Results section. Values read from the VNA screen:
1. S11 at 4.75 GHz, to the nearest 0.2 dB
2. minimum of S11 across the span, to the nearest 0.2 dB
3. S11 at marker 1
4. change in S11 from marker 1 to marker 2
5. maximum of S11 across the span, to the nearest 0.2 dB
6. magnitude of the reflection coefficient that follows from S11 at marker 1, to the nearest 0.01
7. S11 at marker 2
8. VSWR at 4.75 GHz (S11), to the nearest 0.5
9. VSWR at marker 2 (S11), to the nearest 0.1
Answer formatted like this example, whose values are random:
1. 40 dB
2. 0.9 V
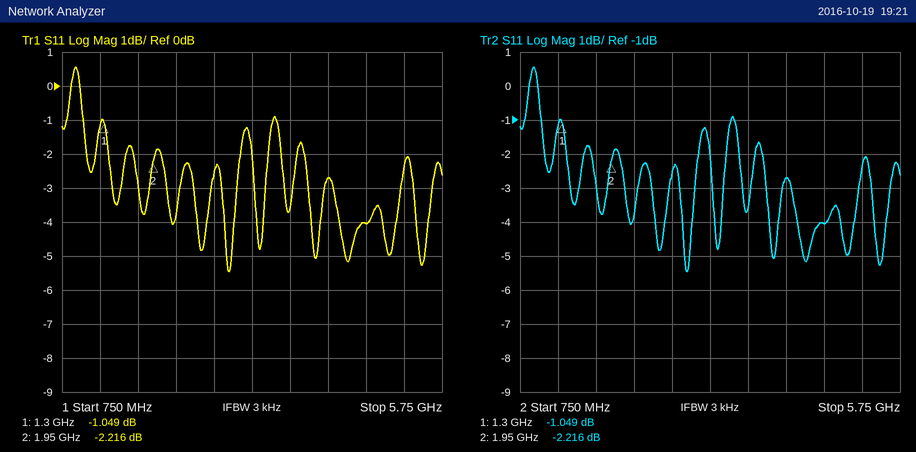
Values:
1. -4.0 dB
2. -5.4 dB
3. -1.049 dB
4. -1.167 dB
5. 0.6 dB
6. 0.89
7. -2.216 dB
8. 4.5
9. 7.9
